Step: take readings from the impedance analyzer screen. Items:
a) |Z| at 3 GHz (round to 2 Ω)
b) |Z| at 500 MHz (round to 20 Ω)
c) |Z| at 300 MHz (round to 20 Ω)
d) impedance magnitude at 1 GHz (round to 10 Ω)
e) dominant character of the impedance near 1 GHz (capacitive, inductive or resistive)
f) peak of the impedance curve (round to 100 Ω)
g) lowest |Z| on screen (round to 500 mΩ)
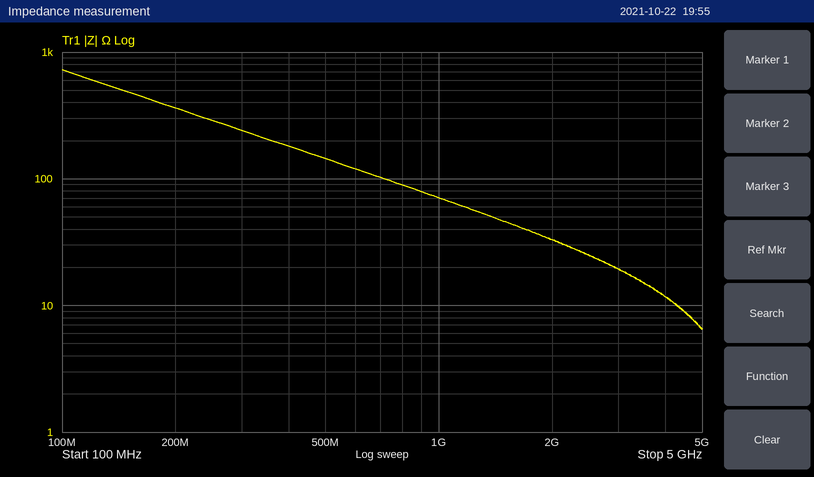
20 Ω
140 Ω
240 Ω
70 Ω
capacitive
700 Ω
6.5 Ω
